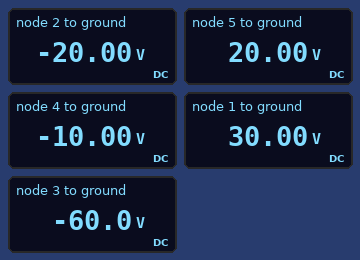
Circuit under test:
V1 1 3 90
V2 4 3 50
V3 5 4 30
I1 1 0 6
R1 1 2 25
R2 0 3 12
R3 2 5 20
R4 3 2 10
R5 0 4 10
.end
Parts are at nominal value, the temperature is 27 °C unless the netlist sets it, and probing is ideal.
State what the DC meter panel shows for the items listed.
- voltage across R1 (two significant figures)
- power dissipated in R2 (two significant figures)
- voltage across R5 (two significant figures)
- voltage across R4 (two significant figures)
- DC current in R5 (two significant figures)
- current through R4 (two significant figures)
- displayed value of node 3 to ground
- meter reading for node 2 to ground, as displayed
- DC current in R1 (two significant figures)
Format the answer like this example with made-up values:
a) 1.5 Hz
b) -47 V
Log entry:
a) 50 V
b) 300 W
c) 10 V
d) 40 V
e) 1.0 A
f) 4.0 A
g) -60.0 V
h) -20.00 V
i) 2.0 A
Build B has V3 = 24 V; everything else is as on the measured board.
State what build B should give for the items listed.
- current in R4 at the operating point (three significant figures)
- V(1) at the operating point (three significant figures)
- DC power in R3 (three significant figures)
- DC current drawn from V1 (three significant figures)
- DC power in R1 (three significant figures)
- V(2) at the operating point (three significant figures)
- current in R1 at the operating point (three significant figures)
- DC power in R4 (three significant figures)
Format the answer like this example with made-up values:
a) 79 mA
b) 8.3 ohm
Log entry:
a) 3.84 A
b) 30.0 V
c) 63.3 W
d) 8.06 A
e) 106 W
f) -21.6 V
g) 2.06 A
h) 148 W
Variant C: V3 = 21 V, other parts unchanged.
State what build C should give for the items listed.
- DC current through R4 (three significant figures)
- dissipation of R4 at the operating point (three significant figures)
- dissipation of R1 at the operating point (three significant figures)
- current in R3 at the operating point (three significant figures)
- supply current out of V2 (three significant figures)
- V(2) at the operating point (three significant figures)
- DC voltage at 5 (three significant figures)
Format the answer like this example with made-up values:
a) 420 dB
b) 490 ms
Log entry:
a) 3.76 A
b) 142 W
c) 110 W
d) 1.67 A
e) 668 mA
f) -22.4 V
g) 11.0 V
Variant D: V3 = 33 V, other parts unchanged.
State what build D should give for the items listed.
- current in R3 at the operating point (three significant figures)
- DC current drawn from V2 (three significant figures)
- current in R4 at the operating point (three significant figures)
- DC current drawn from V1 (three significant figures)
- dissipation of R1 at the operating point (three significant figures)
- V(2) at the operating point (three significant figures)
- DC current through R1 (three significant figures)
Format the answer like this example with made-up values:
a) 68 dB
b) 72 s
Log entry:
a) 2.11 A
b) 1.11 A
c) 4.08 A
d) 7.97 A
e) 96.9 W
f) -19.2 V
g) 1.97 A
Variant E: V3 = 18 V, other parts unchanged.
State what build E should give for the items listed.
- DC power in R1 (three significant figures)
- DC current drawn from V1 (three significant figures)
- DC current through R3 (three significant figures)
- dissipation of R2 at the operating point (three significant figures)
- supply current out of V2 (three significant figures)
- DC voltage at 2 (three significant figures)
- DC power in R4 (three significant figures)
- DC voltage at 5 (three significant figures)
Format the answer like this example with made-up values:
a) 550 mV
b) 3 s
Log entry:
a) 113 W
b) 8.13 A
c) 1.56 A
d) 300 W
e) 558 mA
f) -23.2 V
g) 136 W
h) 8.00 V
